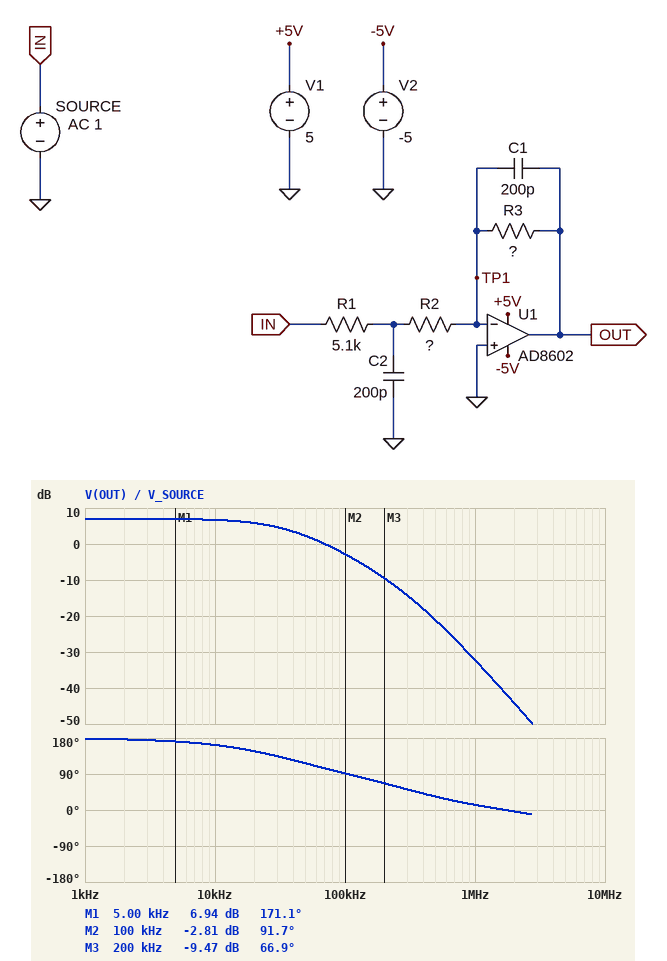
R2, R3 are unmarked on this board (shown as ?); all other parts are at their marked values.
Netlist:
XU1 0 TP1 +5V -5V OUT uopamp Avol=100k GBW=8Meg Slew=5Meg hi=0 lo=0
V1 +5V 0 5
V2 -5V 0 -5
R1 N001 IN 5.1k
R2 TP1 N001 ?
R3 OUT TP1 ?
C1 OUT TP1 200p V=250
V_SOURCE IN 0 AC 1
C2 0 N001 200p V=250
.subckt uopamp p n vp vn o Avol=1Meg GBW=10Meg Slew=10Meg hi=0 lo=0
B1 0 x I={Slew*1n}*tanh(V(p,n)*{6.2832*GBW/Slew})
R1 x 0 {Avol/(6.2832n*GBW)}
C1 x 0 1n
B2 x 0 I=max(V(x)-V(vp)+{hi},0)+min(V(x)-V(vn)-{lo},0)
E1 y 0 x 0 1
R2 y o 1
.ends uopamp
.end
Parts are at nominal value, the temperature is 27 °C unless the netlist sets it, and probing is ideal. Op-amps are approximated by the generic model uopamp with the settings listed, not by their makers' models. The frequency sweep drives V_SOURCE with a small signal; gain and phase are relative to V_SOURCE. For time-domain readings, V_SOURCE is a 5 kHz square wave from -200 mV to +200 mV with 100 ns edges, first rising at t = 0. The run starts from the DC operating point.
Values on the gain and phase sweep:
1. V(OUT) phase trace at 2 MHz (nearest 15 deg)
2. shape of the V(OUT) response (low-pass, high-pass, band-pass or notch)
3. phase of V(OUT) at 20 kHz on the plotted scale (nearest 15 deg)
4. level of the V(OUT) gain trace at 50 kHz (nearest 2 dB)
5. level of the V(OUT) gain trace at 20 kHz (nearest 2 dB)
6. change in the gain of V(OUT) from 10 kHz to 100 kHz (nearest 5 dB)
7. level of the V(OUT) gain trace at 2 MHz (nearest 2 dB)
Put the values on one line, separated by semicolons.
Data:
0 deg; low-pass; 150 deg; 2 dB; 6 dB; -10 dB; -44 dB
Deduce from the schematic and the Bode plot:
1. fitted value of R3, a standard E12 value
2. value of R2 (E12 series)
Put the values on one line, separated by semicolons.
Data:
22 kΩ; 4.7 kΩ
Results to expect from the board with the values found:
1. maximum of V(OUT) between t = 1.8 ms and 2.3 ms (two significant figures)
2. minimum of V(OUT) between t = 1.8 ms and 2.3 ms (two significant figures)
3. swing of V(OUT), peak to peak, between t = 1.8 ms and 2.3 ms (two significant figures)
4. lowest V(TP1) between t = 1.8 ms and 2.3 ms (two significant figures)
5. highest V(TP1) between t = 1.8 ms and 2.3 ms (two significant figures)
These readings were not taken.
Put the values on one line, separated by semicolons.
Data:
450 mV; -450 mV; 900 mV; -3.1 mV; 3.1 mV
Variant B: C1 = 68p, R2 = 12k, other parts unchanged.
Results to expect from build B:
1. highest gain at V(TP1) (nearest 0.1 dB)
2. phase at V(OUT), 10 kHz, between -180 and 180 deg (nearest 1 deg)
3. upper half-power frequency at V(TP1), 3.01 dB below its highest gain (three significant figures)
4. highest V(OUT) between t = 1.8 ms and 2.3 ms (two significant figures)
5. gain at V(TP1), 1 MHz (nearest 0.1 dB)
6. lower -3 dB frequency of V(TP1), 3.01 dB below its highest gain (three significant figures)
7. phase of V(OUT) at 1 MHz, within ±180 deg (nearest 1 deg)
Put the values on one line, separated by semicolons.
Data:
-38.8 dB; 172 deg; 384 kHz; 260 mV; -48.9 dB; 60.0 kHz; 11 deg
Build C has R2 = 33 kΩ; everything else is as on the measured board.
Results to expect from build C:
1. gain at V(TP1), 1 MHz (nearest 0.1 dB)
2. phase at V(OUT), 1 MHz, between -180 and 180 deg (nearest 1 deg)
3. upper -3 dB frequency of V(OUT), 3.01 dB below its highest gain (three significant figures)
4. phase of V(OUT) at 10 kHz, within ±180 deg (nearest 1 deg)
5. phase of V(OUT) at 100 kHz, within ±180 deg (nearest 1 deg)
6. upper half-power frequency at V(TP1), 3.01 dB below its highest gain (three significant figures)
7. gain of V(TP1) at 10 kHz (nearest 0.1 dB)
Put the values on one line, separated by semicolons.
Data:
-66.8 dB; 5 deg; 34.8 kHz; 161 deg; 80 deg; 243 kHz; -63.2 dB
